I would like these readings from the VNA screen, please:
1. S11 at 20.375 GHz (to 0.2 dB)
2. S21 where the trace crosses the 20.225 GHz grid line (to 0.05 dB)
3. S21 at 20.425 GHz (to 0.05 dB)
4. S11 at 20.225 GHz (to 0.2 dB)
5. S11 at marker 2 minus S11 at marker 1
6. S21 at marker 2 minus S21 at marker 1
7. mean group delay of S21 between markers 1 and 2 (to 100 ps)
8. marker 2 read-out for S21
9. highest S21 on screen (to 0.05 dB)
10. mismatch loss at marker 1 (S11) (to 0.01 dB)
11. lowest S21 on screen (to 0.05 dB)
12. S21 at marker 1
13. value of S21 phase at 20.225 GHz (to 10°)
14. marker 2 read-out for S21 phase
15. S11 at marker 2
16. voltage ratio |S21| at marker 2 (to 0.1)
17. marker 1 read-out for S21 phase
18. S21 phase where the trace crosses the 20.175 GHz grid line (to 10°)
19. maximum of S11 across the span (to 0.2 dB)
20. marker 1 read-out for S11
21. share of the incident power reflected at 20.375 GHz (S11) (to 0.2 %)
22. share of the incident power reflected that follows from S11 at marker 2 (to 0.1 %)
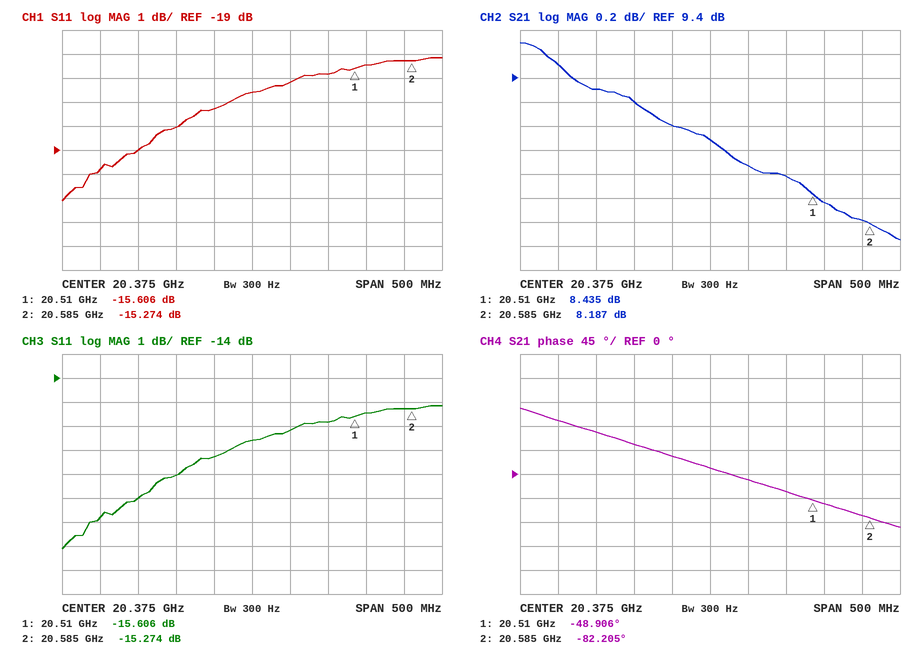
-16.6 dB
9.30 dB
8.65 dB
-19.0 dB
0.332 dB
-0.248 dB
1.2 ns
8.187 dB
9.70 dB
0.12 dB
8.05 dB
8.435 dB
80°
-82.205°
-15.274 dB
2.6
-48.906°
100°
-15.2 dB
-15.606 dB
2.2 %
3.0 %
